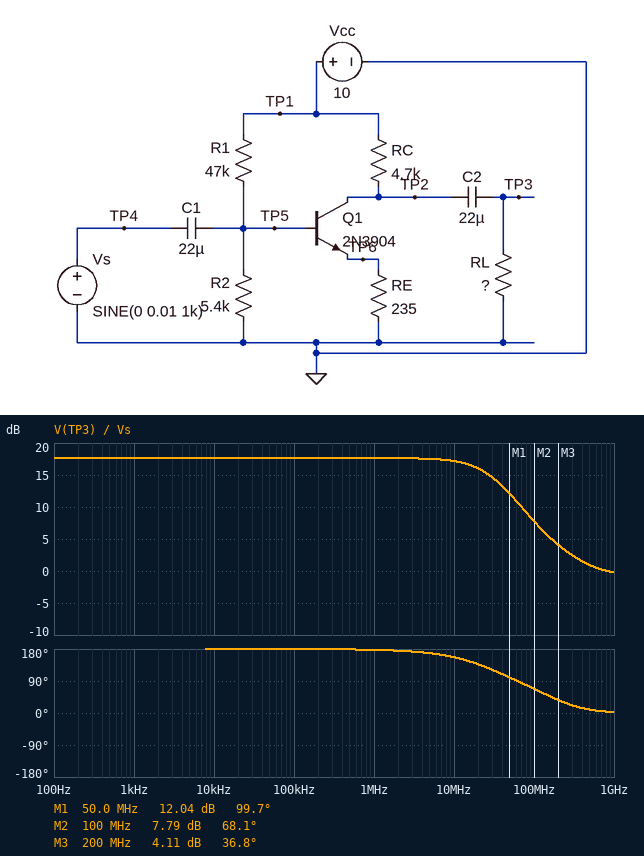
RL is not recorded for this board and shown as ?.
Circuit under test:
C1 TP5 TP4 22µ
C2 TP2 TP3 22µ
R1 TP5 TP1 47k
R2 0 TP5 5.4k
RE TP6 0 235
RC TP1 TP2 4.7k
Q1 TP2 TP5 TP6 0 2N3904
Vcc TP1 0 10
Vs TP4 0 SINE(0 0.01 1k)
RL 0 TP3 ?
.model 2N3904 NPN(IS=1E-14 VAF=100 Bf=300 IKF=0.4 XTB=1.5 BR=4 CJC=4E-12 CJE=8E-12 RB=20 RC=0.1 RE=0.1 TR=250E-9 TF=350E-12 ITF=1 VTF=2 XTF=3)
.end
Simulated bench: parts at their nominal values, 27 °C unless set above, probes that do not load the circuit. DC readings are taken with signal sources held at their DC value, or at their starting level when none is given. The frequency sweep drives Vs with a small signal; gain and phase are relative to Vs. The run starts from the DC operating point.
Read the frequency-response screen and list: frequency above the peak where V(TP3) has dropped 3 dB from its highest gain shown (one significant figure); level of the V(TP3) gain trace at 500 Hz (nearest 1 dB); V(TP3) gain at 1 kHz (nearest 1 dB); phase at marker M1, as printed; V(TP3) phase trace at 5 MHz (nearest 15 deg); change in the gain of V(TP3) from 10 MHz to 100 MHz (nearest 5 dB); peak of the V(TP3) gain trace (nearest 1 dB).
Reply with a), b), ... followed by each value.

a) 30 MHz
b) 18 dB
c) 18 dB
d) 99.7 deg
e) 165 deg
f) -10 dB
g) 18 dB
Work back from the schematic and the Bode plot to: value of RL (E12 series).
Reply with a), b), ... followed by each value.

a) 3.3 kΩ
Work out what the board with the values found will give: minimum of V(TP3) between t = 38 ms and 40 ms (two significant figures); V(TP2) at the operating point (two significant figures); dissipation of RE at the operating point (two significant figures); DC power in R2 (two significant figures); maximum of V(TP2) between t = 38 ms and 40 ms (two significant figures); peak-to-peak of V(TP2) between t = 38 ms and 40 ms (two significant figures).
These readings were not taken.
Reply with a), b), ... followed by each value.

a) -76 mV
b) 3.2 V
c) 500 µW
d) 190 µW
e) 3.2 V
f) 150 mV
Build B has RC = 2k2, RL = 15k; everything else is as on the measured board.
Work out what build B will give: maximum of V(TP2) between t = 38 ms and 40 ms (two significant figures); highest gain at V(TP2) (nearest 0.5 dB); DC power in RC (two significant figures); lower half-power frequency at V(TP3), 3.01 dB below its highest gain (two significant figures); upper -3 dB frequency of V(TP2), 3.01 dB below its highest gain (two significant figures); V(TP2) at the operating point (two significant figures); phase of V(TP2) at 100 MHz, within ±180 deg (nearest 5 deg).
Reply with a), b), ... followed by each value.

a) 6.9 V
b) 17.5 dB
c) 4.7 mW
d) 1.7 Hz
e) 40 MHz
f) 6.8 V
g) 75 deg
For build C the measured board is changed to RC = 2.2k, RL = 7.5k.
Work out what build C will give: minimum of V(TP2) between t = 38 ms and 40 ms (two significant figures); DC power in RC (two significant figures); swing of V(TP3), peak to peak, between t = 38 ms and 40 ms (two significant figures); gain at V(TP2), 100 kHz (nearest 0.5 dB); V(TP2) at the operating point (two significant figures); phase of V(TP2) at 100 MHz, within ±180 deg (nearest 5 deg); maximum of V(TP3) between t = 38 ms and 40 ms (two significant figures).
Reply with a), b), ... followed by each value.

a) 6.7 V
b) 4.7 mW
c) 130 mV
d) 16.5 dB
e) 6.8 V
f) 80 deg
g) 67 mV
